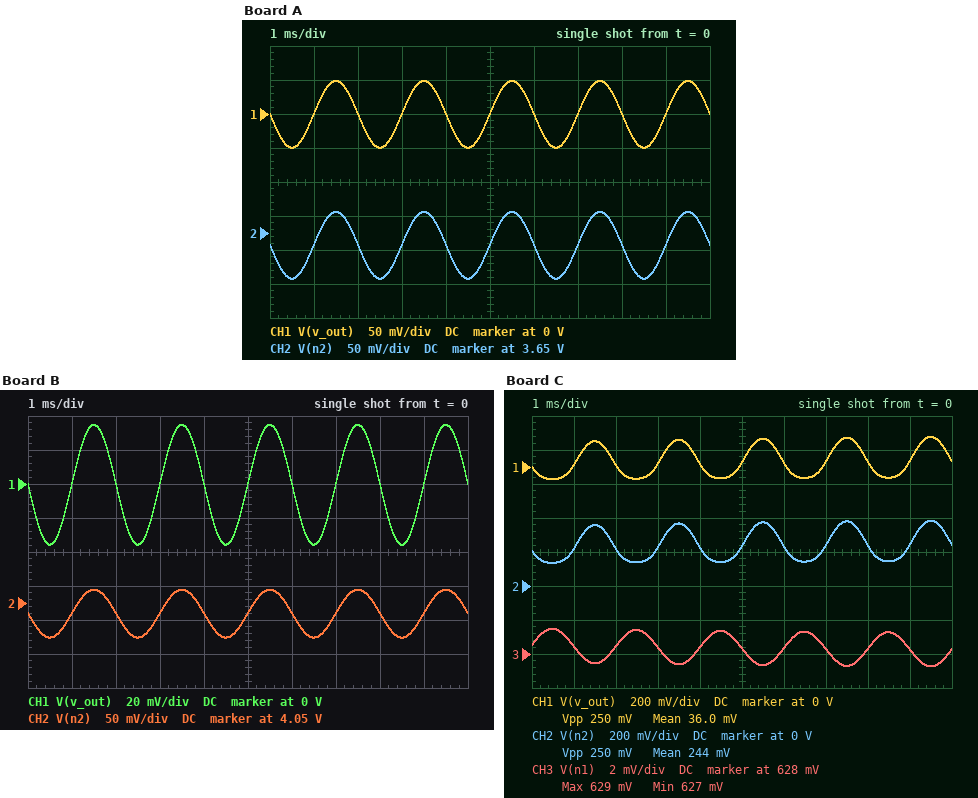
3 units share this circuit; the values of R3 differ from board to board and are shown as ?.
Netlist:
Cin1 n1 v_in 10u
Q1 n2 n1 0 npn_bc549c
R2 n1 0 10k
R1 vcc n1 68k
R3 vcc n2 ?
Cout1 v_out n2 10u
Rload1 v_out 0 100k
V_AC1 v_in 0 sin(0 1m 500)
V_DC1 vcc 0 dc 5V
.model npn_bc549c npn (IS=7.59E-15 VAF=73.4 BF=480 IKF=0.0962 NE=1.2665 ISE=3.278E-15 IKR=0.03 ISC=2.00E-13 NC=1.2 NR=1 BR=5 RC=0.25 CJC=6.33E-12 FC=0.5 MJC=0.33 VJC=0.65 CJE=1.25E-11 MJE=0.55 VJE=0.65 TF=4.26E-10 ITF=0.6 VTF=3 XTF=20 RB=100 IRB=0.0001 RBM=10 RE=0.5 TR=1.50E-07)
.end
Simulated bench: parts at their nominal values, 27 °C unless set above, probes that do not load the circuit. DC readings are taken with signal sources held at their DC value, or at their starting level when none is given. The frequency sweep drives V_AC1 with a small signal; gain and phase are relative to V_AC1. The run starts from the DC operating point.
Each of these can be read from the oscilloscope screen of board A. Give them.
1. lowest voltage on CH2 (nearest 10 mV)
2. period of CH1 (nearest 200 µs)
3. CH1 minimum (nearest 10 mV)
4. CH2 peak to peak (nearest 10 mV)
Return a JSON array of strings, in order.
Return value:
["3.58 V", "2.0 ms", "-50 mV", "100 mV"]
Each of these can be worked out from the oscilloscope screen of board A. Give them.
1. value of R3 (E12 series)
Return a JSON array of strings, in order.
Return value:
["4.7 kΩ"]
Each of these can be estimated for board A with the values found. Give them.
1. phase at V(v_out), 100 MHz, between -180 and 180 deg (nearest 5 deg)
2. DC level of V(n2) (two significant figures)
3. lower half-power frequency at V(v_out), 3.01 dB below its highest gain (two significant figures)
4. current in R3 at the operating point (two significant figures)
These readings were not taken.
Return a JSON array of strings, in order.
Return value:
["40 deg", "3.6 V", "2.5 Hz", "290 µA"]
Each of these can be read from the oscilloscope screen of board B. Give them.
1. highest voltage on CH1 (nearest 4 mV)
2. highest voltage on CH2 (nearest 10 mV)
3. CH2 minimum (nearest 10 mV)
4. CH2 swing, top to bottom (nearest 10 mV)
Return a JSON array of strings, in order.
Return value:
["36 mV", "4.07 V", "4.00 V", "70 mV"]
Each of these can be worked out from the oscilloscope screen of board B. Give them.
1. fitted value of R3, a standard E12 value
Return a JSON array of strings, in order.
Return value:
["3.3 kΩ"]
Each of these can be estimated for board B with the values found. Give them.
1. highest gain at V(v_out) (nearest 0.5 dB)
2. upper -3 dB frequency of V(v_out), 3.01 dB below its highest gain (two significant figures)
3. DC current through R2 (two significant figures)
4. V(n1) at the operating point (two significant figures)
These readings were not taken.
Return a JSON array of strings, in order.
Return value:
["31.0 dB", "6.4 MHz", "63 µA", "630 mV"]
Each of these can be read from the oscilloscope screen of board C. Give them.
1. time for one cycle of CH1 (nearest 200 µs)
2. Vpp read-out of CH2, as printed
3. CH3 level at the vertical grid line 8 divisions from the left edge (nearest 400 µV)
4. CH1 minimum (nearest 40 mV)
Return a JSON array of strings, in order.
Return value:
["2.0 ms", "250 mV", "628.4 mV", "-80 mV"]
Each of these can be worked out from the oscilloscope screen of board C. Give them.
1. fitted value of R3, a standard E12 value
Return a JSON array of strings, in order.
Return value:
["18 kΩ"]
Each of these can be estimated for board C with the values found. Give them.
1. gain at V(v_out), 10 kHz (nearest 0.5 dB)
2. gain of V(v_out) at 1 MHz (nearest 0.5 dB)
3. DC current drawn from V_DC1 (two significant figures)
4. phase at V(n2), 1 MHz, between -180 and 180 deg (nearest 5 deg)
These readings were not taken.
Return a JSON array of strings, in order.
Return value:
["41.5 dB", "37.0 dB", "330 µA", "125 deg"]
